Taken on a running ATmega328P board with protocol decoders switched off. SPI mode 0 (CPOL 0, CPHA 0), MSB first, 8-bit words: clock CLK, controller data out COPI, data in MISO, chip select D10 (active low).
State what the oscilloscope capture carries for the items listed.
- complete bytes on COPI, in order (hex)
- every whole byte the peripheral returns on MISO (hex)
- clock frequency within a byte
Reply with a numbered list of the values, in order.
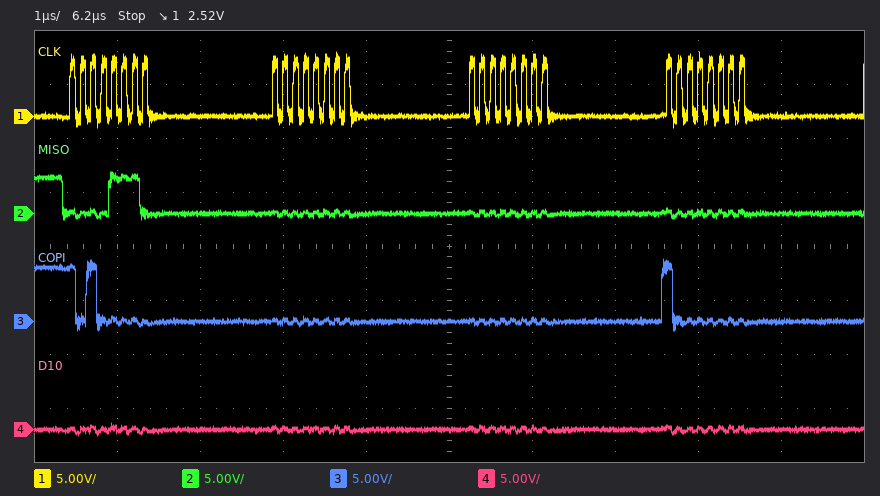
1. A0 00 00 80
2. 0E 00 00 00
3. 8 MHz
